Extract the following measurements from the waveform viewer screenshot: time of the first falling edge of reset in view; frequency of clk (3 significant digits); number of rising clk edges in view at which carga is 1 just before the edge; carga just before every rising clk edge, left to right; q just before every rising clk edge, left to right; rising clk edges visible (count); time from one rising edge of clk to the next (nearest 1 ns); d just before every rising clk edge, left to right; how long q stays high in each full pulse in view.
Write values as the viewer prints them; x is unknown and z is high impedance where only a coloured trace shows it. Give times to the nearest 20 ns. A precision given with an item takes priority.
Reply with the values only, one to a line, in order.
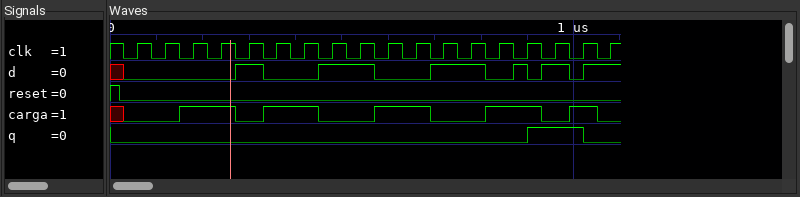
20 ns
16.7 MHz
9
0 0 1 1 0 1 1 0 0 1 1 0 0 1 1 0 1 0
0 0 0 0 0 0 0 0 0 0 0 0 0 0 0 1 1 0
18
60 ns
0 0 0 0 1 0 0 1 1 0 0 1 1 0 1 1 0 1
120 ns
